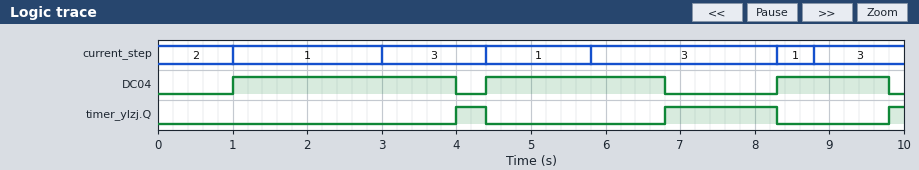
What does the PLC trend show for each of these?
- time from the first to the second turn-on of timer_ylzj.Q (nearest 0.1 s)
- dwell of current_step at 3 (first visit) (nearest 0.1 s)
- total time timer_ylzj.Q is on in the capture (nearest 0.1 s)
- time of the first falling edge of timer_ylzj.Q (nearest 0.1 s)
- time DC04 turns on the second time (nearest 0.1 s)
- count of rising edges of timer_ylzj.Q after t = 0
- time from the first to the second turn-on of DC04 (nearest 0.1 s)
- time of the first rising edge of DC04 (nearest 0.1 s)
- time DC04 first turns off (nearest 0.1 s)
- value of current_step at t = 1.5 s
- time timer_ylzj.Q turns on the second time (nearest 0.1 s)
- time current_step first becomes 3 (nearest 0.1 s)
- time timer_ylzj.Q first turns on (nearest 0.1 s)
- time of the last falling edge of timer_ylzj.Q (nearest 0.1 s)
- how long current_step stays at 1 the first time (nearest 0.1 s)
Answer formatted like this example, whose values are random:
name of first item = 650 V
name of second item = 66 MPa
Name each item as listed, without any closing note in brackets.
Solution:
time from the first to the second turn-on of timer_ylzj.Q = 2.8 s
dwell of current_step at 3 (first visit) = 1.4 s
total time timer_ylzj.Q is on in the capture = 2.1 s
time of the first falling edge of timer_ylzj.Q = 4.4 s
time DC04 turns on the second time = 4.4 s
count of rising edges of timer_ylzj.Q after t = 0 = 3
time from the first to the second turn-on of DC04 = 3.4 s
time of the first rising edge of DC04 = 1.0 s
time DC04 first turns off = 4.0 s
value of current_step at t = 1.5 s = 1
time timer_ylzj.Q turns on the second time = 6.8 s
time current_step first becomes 3 = 3.0 s
time timer_ylzj.Q first turns on = 4.0 s
time of the last falling edge of timer_ylzj.Q = 8.3 s
how long current_step stays at 1 the first time = 2.0 s
